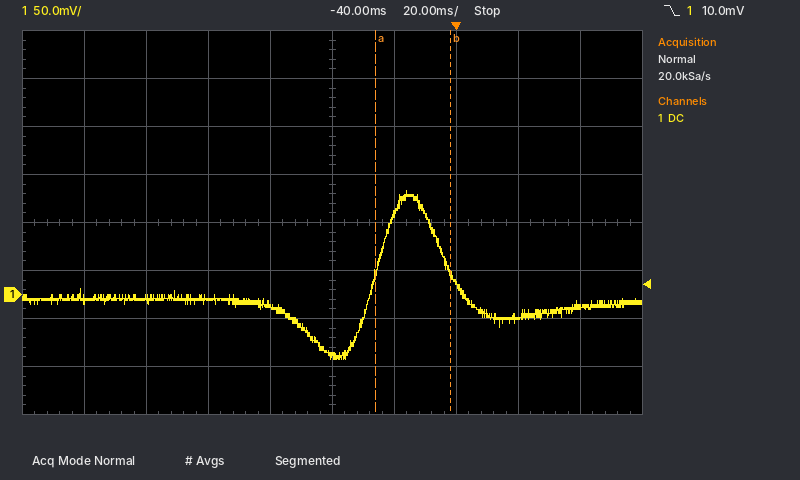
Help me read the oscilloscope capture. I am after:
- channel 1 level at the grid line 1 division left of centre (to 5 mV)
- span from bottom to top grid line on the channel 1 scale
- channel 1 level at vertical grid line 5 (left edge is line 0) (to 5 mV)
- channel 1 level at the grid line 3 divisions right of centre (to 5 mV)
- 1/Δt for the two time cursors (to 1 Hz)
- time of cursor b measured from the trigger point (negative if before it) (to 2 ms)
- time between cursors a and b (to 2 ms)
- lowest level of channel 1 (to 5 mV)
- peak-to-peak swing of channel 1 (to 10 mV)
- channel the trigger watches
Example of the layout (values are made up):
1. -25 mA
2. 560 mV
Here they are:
1. -10 mV
2. 400 mV
3. -65 mV
4. -25 mV
5. 42 Hz
6. -2 ms
7. 24 ms
8. -70 mV
9. 180 mV
10. channel 1
